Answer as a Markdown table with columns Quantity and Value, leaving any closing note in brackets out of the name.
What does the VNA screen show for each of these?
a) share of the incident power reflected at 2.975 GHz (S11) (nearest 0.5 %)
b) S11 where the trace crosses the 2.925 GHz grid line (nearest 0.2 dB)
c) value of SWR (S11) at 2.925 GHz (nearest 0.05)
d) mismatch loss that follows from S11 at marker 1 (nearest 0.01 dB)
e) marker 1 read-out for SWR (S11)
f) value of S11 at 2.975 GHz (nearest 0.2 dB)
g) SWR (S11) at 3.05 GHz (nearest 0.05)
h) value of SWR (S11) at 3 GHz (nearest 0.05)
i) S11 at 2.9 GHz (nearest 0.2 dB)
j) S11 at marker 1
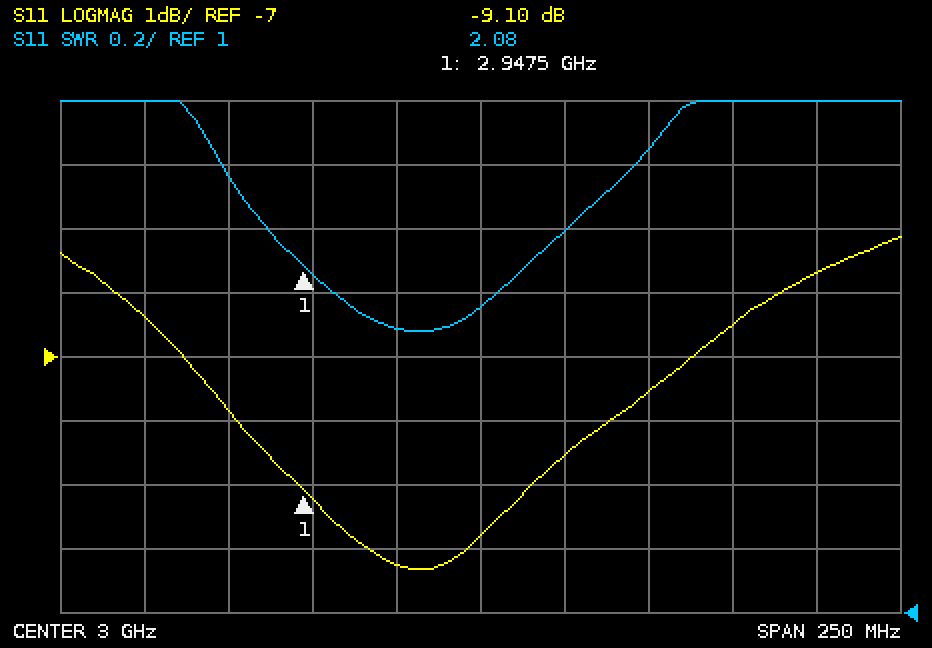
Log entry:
| Quantity | Value |
|---|---|
| share of the incident power reflected at 2.975 GHz (S11) | 9.5 % |
| S11 where the trace crosses the 2.925 GHz grid line | -7.8 dB |
| value of SWR (S11) at 2.925 GHz | 2.35 |
| mismatch loss that follows from S11 at marker 1 | 0.57 dB |
| marker 1 read-out for SWR | 2.08 |
| value of S11 at 2.975 GHz | -10.2 dB |
| SWR (S11) at 3.05 GHz | 2.45 |
| value of SWR (S11) at 3 GHz | 1.95 |
| S11 at 2.9 GHz | -6.4 dB |
| S11 at marker 1 | -9.10 dB |
